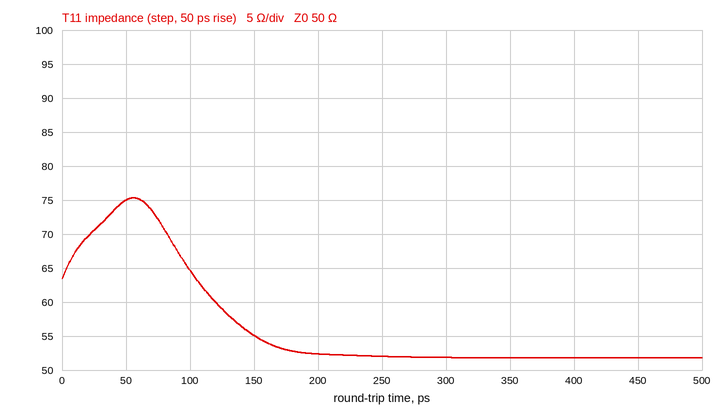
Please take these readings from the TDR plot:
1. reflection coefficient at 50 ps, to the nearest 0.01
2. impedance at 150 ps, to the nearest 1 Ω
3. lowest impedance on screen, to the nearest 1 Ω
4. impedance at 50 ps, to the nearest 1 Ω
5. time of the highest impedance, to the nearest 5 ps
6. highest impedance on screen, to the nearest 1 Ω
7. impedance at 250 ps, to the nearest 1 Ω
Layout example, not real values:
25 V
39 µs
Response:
+0.20
55 Ω
52 Ω
75 Ω
55 ps
75 Ω
52 Ω
